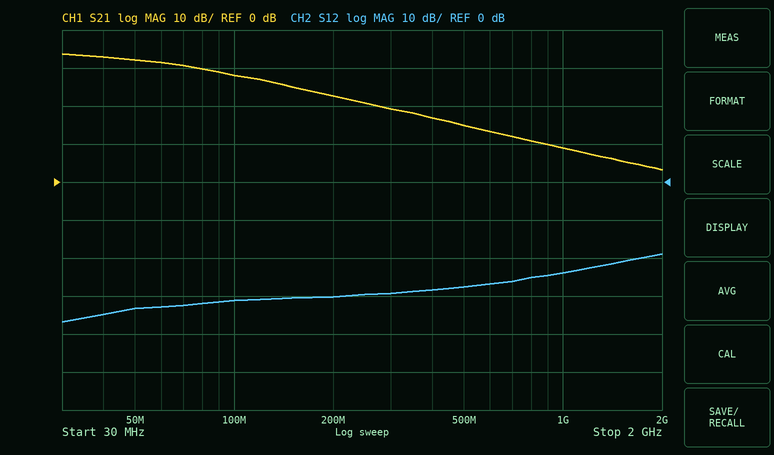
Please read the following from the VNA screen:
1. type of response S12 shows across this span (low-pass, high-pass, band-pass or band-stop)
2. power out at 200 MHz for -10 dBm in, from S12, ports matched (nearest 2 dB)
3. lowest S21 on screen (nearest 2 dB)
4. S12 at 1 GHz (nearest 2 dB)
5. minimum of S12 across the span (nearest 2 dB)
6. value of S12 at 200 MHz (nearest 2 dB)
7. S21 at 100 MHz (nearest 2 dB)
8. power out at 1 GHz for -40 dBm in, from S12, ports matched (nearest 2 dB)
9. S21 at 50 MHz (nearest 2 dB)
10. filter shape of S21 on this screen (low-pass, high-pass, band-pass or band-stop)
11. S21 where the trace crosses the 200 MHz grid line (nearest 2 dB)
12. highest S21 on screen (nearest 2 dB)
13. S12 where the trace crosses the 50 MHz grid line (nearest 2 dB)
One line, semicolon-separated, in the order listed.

high-pass; -40 dBm; 4 dB; -24 dB; -36 dB; -30 dB; 28 dB; -64 dBm; 32 dB; low-pass; 22 dB; 34 dB; -34 dB
